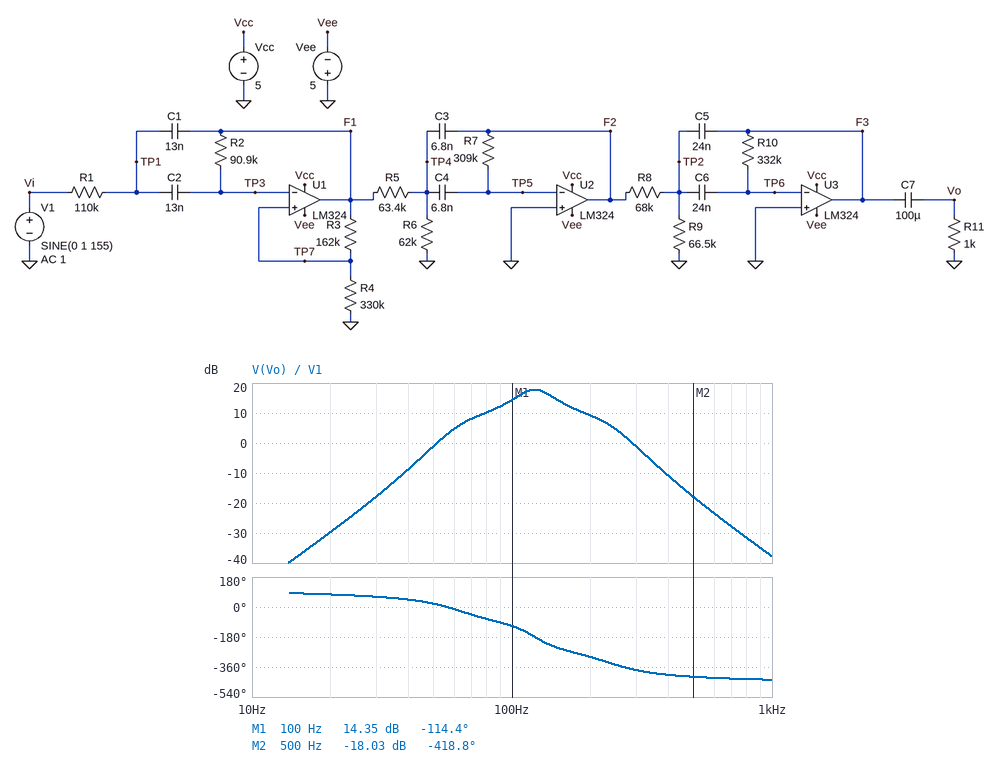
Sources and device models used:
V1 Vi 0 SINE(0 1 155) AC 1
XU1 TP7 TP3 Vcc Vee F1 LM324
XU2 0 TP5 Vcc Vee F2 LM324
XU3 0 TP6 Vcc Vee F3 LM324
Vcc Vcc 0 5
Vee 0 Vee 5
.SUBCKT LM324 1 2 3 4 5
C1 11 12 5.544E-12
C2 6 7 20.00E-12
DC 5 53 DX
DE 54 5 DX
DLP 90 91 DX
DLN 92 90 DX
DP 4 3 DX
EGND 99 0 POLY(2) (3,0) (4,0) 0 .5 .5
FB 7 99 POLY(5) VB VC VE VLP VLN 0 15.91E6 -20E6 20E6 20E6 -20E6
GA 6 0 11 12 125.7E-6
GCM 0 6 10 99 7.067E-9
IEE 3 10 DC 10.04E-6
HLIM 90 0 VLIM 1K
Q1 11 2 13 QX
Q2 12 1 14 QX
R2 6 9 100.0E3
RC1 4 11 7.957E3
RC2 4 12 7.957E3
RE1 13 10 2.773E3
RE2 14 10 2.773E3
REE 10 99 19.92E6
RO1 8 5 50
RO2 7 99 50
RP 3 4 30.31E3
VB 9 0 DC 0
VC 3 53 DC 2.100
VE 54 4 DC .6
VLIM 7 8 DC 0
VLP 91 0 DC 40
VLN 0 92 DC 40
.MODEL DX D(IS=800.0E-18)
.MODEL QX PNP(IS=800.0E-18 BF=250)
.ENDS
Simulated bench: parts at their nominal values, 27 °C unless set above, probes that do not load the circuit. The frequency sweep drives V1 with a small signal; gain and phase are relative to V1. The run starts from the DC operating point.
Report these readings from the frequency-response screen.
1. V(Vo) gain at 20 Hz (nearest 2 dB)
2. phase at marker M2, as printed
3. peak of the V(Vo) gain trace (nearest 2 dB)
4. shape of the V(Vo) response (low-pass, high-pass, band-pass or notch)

-30 dB
-418.8 deg
18 dB
band-pass
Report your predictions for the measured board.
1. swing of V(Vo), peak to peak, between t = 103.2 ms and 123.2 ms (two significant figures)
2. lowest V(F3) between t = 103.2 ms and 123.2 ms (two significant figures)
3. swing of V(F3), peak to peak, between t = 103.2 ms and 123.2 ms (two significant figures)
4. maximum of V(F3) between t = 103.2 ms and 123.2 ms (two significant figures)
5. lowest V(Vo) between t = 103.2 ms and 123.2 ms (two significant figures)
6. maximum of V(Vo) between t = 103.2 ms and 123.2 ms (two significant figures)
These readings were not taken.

6.9 V
-3.4 V
6.9 V
3.5 V
-3.4 V
3.5 V
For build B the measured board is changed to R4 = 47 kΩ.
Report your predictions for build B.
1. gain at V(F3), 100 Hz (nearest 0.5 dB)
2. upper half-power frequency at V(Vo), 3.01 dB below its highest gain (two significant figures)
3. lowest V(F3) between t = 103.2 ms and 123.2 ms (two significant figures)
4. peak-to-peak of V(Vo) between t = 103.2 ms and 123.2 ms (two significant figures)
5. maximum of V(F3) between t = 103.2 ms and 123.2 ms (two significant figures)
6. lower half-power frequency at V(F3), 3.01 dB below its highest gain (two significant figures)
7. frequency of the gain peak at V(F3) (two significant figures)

-4.5 dB
260 Hz
-610 mV
1.2 V
600 mV
58 Hz
180 Hz
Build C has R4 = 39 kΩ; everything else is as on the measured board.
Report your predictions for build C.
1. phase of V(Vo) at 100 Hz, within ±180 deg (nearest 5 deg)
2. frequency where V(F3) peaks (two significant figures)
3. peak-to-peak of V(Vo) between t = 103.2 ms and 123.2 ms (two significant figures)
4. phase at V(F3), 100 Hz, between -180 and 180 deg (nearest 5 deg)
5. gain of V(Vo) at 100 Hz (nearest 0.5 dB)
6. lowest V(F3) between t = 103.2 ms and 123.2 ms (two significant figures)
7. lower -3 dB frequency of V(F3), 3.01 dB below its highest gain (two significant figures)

-150 deg
180 Hz
1.1 V
-155 deg
-5.0 dB
-570 mV
58 Hz
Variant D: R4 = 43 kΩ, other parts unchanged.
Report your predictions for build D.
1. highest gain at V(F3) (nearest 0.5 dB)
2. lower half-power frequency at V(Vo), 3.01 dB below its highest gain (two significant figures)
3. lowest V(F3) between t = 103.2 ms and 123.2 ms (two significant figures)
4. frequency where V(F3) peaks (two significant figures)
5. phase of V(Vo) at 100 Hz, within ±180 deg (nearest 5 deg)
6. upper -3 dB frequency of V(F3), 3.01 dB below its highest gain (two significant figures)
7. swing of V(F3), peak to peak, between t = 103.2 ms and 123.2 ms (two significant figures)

-4.5 dB
58 Hz
-590 mV
180 Hz
-150 deg
260 Hz
1.2 V
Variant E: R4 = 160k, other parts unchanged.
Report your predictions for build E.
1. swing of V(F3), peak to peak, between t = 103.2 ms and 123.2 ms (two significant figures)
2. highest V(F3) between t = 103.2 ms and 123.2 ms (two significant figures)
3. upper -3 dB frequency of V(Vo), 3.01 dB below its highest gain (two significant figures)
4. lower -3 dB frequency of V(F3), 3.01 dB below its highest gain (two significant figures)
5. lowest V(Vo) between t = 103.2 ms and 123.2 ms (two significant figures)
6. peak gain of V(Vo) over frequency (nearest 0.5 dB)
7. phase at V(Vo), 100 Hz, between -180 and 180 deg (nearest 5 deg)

2.7 V
1.3 V
240 Hz
62 Hz
-1.3 V
2.5 dB
-145 deg
